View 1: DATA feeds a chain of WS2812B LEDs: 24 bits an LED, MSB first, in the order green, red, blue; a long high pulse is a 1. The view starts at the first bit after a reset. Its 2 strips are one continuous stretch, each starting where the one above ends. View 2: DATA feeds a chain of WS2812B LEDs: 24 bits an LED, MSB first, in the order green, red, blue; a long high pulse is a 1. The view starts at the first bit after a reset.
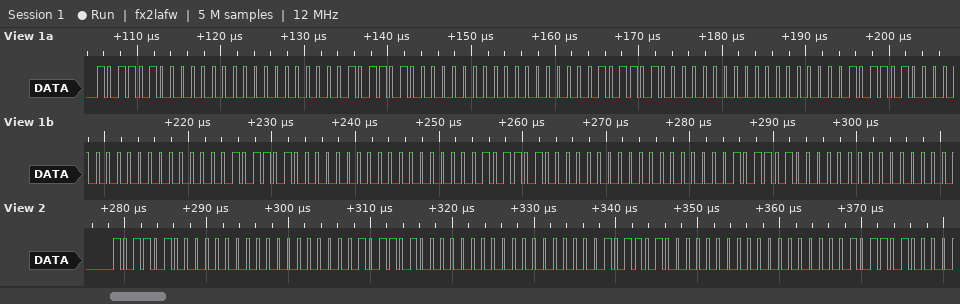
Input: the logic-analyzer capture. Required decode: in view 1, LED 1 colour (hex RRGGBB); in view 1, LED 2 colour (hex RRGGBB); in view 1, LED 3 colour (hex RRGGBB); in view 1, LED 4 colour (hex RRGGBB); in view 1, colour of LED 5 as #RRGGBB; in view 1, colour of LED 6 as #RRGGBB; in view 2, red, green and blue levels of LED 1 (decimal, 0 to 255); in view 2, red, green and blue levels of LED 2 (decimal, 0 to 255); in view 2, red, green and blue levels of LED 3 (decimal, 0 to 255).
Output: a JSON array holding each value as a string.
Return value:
["#00B400", "#00B400", "#00B400", "#00B400", "#00B400", "#00B400", "0, 180, 0", "0, 180, 0", "0, 180, 0"]
